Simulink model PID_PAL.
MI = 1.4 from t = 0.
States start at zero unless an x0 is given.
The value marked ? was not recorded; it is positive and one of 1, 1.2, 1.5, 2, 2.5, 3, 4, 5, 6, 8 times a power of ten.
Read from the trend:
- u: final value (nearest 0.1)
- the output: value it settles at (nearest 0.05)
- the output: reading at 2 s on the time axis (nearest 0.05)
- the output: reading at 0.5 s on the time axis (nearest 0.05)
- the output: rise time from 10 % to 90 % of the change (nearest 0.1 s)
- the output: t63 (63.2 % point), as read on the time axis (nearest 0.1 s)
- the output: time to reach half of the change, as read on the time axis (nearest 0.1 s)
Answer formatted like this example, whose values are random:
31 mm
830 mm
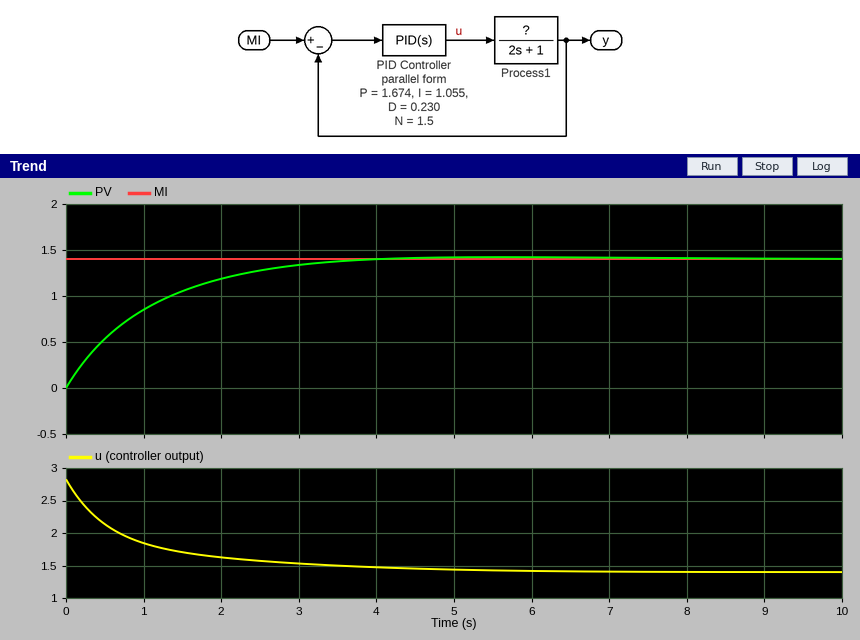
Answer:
1.4
1.40
1.20
0.55
2.3 s
1.1 s
0.7 s
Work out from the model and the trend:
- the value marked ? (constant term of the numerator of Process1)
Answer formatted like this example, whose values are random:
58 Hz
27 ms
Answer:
1
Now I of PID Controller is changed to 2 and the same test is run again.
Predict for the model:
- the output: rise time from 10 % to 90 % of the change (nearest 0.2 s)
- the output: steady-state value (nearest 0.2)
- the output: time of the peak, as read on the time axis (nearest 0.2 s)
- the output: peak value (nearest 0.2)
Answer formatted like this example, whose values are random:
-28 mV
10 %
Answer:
1.4 s
1.4
3.2 s
1.6
